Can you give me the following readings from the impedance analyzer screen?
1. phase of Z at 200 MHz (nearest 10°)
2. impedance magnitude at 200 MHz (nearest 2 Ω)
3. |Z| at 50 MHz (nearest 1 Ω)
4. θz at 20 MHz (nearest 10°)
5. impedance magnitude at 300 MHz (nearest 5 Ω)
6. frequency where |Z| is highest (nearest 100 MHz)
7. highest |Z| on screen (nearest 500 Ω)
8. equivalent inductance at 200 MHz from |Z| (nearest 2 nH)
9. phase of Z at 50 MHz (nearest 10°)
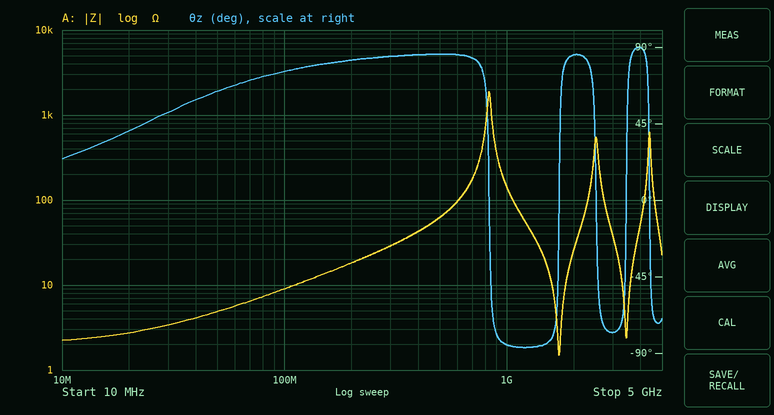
80°
18 Ω
5 Ω
40°
30 Ω
800 MHz
2.0 kΩ
14 nH
60°
